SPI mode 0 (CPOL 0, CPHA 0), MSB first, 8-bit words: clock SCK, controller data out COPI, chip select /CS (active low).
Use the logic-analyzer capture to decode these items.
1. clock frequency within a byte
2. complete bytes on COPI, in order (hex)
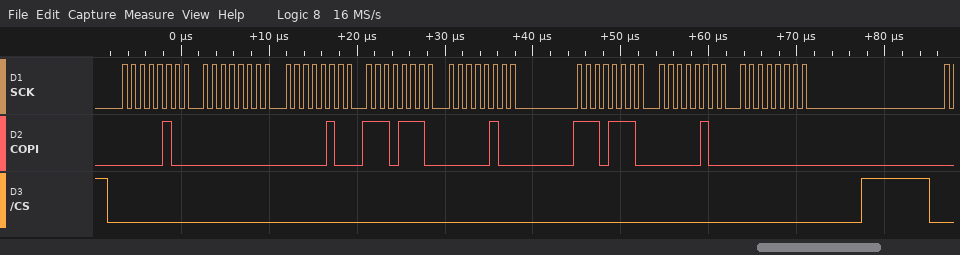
1 MHz
0x04 0x00 0x04 0xEE 0x04 0xEE 0x04 0x00
